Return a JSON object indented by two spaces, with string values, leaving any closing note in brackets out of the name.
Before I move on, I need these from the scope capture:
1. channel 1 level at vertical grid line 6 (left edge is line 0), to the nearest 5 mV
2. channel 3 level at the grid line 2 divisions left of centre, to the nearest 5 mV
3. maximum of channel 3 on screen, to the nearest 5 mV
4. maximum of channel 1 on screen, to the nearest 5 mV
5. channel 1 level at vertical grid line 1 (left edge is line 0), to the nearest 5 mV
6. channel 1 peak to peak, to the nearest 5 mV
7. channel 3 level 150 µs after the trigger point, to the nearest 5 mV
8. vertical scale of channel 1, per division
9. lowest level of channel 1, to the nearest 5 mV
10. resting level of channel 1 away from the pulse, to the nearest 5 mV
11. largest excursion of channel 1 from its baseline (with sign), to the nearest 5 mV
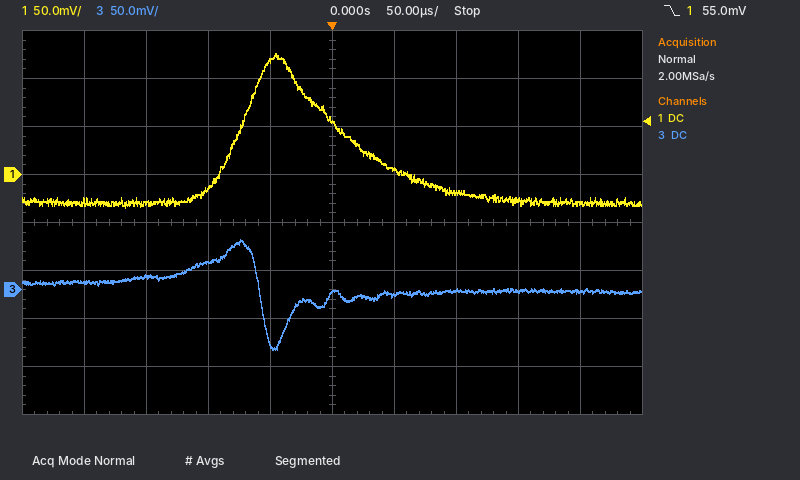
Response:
{
  "channel 1 level at vertical grid line 6 (left edge is line 0), to the nearest 5 mV": "5 mV",
  "channel 3 level at the grid line 2 divisions left of centre, to the nearest 5 mV": "30 mV",
  "maximum of channel 3 on screen, to the nearest 5 mV": "50 mV",
  "maximum of channel 1 on screen, to the nearest 5 mV": "125 mV",
  "channel 1 level at vertical grid line 1 (left edge is line 0), to the nearest 5 mV": "-30 mV",
  "channel 1 peak to peak, to the nearest 5 mV": "160 mV",
  "channel 3 level 150 µs after the trigger point, to the nearest 5 mV": "0 mV",
  "vertical scale of channel 1, per division": "50 mV",
  "lowest level of channel 1, to the nearest 5 mV": "-35 mV",
  "resting level of channel 1 away from the pulse, to the nearest 5 mV": "-30 mV",
  "largest excursion of channel 1 from its baseline (with sign), to the nearest 5 mV": "+155 mV"
}
